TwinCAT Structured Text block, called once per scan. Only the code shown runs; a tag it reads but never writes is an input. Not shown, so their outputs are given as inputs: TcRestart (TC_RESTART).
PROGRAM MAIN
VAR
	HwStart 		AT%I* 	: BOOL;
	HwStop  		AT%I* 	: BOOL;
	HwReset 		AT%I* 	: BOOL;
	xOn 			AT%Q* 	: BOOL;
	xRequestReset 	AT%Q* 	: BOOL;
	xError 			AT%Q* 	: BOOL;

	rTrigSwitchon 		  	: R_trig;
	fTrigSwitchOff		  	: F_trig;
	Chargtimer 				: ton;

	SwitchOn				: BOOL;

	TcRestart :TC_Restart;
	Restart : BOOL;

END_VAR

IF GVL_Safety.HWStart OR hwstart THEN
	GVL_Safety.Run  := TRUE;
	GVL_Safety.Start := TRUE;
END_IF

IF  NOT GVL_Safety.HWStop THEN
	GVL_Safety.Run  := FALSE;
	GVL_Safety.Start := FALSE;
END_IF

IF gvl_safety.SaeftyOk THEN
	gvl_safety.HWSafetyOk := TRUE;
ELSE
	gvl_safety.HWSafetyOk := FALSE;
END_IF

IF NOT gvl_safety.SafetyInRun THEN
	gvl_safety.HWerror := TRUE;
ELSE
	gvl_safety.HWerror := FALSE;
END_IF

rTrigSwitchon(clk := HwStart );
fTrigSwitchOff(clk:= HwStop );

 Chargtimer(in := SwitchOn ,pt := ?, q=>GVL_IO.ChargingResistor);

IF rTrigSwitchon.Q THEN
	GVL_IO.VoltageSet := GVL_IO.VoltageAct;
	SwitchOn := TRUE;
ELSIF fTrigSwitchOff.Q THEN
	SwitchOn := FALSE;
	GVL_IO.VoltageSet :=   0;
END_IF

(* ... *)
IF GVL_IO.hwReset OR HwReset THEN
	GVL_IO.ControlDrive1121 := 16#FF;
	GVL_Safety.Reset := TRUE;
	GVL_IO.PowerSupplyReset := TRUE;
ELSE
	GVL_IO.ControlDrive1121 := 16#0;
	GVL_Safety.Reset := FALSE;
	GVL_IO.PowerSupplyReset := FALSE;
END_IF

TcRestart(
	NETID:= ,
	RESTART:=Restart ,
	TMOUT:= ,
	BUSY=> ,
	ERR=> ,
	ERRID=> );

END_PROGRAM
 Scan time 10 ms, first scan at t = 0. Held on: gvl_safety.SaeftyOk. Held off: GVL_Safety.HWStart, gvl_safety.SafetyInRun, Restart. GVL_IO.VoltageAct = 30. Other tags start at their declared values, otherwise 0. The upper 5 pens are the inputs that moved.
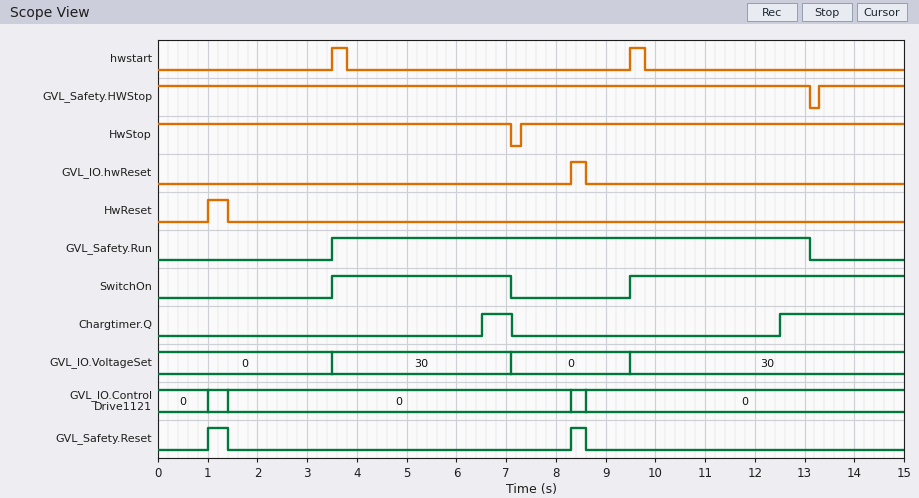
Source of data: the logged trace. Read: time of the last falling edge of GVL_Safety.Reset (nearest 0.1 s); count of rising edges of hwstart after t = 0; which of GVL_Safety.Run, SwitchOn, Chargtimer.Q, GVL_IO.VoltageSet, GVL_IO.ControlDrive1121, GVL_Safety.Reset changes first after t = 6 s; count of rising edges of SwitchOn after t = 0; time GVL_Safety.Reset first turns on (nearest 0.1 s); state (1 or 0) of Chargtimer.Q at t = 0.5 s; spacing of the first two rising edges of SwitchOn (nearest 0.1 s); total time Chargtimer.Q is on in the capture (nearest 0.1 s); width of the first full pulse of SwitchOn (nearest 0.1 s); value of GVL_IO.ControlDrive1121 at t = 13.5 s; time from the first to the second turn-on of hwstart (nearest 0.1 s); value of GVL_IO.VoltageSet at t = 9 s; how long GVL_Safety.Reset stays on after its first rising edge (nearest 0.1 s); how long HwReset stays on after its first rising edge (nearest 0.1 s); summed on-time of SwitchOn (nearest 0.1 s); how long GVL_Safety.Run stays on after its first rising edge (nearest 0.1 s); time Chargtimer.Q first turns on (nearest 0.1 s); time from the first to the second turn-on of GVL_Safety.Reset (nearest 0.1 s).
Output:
8.6 s
2
Chargtimer.Q
2
1.0 s
0
6.0 s
3.1 s
3.6 s
0
6.0 s
0
0.4 s
0.4 s
9.1 s
9.6 s
6.5 s
7.3 s
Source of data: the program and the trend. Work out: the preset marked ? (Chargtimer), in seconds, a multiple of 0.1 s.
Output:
3.0 s
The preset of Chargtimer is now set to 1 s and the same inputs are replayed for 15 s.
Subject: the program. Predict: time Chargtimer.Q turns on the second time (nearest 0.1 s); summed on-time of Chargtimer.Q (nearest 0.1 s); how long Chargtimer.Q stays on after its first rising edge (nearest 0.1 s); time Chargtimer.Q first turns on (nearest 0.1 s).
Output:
10.5 s
7.1 s
2.6 s
4.5 s
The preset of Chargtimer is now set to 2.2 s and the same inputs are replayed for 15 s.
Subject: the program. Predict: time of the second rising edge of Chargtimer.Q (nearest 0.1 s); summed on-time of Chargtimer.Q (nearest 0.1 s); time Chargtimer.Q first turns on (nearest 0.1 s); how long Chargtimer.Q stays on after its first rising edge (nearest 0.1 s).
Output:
11.7 s
4.7 s
5.7 s
1.4 s
